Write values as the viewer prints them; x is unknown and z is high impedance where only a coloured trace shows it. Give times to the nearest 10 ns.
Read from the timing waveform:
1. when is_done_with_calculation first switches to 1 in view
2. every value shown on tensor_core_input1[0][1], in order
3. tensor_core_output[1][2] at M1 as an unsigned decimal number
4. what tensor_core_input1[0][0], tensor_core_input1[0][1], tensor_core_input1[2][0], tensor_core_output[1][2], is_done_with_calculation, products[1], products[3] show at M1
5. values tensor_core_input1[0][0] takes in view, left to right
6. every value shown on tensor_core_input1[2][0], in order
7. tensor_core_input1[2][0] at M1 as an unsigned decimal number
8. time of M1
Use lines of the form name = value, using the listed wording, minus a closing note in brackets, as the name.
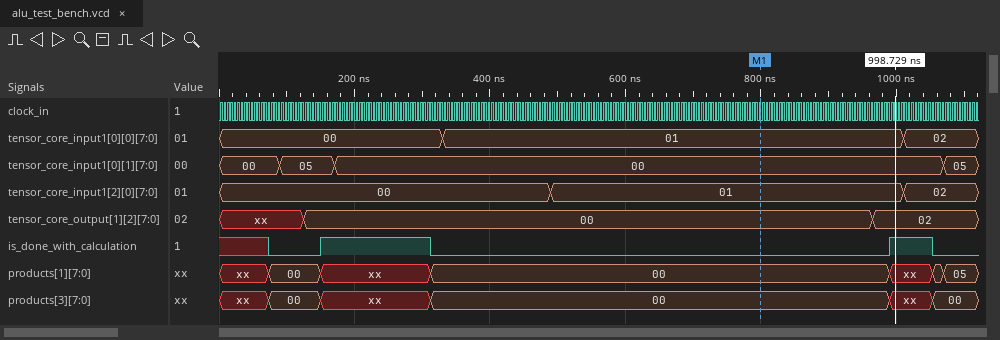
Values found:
when is_done_with_calculation first switches to 1 in view = 150 ns
every value shown on tensor_core_input1[0][1], in order = 00, 05, 00, 05
tensor_core_output[1][2] at M1 as an unsigned decimal number = 0
what tensor_core_input1[0][0], tensor_core_input1[0][1], tensor_core_input1[2][0], tensor_core_output[1][2], is_done_with_calculation, products[1], products[3] show at M1 = tensor_core_input1[0][0]=01, tensor_core_input1[0][1]=00, tensor_core_input1[2][0]=01, tensor_core_output[1][2]=00, is_done_with_calculation=0, products[1]=00, products[3]=00
values tensor_core_input1[0][0] takes in view, left to right = 00, 01, 02
every value shown on tensor_core_input1[2][0], in order = 00, 01, 02
tensor_core_input1[2][0] at M1 as an unsigned decimal number = 1
time of M1 = 800 ns
